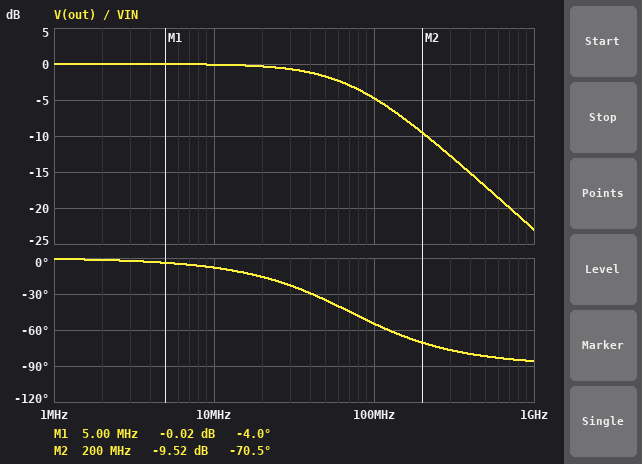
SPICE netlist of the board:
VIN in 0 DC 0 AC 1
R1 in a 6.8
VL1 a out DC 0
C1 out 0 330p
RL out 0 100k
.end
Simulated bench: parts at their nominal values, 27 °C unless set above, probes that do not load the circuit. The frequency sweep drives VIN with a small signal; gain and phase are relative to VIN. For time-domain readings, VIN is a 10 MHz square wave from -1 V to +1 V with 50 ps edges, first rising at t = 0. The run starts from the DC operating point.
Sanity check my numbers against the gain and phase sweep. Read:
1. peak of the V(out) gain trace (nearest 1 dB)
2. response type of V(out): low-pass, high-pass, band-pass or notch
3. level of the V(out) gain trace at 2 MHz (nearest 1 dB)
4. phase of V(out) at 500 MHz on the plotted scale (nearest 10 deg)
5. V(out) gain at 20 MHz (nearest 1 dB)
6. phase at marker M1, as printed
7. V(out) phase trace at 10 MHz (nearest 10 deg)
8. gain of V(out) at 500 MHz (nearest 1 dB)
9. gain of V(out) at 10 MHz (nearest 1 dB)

0 dB
low-pass
0 dB
-80 deg
0 dB
-4.0 deg
-10 deg
-17 dB
0 dB
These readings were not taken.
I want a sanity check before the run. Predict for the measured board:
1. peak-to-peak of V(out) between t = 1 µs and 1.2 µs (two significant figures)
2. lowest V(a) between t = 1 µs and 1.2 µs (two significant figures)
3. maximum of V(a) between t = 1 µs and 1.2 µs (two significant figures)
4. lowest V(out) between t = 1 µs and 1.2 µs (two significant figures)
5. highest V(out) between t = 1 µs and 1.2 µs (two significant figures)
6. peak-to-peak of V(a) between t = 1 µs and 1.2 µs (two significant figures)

2.0 V
-1.0 V
1.0 V
-1.0 V
1.0 V
2.0 V
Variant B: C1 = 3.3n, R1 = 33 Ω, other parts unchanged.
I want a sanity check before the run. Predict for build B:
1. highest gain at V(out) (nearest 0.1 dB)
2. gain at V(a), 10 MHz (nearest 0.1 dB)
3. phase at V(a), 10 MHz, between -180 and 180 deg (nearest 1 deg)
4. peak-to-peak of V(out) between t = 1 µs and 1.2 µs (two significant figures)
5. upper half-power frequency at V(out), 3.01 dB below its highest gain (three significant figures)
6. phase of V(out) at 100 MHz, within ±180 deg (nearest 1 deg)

0 dB
-16.8 dB
-82 deg
450 mV
1.46 MHz
-89 deg
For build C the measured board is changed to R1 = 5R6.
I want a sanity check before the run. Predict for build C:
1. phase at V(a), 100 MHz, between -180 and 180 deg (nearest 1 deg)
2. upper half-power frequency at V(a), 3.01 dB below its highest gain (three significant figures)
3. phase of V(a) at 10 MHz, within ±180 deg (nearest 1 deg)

-49 deg
86.1 MHz
-7 deg
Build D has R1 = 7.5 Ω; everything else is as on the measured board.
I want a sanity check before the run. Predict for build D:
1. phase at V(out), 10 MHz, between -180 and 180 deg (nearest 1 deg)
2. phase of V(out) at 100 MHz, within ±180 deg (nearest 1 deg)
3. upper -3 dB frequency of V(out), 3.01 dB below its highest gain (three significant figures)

-9 deg
-57 deg
64.3 MHz
